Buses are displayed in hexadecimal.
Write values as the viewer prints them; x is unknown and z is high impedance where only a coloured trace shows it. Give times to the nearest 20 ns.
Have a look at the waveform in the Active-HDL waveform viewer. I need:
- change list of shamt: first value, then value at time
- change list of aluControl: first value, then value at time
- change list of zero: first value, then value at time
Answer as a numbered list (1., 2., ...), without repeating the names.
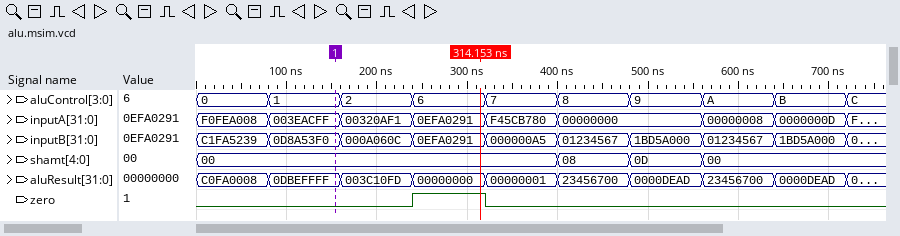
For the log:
1. 00, 08 at 400 ns, 0D at 480 ns, 00 at 560 ns
2. 0, 1 at 80 ns, 2 at 160 ns, 6 at 240 ns, 7 at 320 ns, 8 at 400 ns, 9 at 480 ns, A at 560 ns, B at 640 ns, C at 720 ns
3. 0, 1 at 240 ns, 0 at 320 ns
